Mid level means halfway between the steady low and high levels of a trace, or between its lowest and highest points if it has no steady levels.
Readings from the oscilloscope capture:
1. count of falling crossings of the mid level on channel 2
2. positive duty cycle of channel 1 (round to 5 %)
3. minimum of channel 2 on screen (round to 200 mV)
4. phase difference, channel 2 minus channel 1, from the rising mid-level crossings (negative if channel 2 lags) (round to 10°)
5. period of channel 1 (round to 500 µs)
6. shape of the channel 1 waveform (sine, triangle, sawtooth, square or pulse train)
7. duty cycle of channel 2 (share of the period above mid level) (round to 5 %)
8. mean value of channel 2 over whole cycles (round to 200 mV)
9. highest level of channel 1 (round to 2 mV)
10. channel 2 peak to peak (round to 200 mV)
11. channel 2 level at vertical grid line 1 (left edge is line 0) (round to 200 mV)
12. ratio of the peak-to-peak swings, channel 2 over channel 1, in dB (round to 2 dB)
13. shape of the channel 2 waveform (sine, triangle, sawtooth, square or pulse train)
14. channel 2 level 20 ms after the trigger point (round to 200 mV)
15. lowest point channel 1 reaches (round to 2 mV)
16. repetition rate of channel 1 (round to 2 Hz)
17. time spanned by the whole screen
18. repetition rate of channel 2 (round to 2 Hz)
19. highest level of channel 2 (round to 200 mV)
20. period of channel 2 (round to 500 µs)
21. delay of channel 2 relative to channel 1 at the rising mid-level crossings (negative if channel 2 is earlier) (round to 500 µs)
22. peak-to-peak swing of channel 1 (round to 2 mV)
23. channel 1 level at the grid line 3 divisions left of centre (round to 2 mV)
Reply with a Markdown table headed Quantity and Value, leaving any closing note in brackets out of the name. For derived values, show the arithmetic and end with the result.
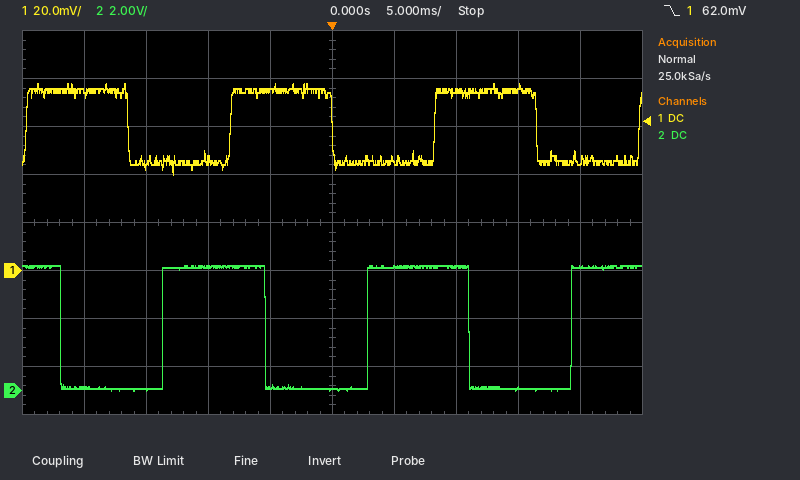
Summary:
| Quantity | Value |
|---|---|
| count of falling crossings of the mid level on channel 2 | 3 |
| positive duty cycle of channel 1 | 50 % |
| minimum of channel 2 on screen | 0.0 V |
| phase difference, channel 2 minus channel 1, from the rising mid-level crossings (negative if channel 2 lags) | −360° × (-5.5 ms) / 16.5 ms ≈ +120° |
| period of channel 1 | 16.5 ms |
| shape of the channel 1 waveform | square |
| duty cycle of channel 2 (share of the period above mid level) | 50 % |
| mean value of channel 2 over whole cycles | 0.0 V + 0.5 × (5.2 V − (0.0 V)) ≈ 2.6 V |
| highest level of channel 1 | 78 mV |
| channel 2 peak to peak | 5.2 V − (0.0 V) = 5.2 V |
| channel 2 level at vertical grid line 1 (left edge is line 0) | 200 mV |
| ratio of the peak-to-peak swings, channel 2 over channel 1, in dB | 20 log10(5.2 V / 38 mV) ≈ 42.7 dB, so 42 dB to the nearest 2 dB |
| shape of the channel 2 waveform | square |
| channel 2 level 20 ms after the trigger point | 5.2 V |
| lowest point channel 1 reaches | 40 mV |
| repetition rate of channel 1 | 1 / 16.5 ms ≈ 60.6 Hz, so 60 Hz to the nearest 2 Hz |
| time spanned by the whole screen | 50 ms |
| repetition rate of channel 2 | 1 / 16.5 ms ≈ 60.6 Hz, so 60 Hz to the nearest 2 Hz |
| highest level of channel 2 | 5.2 V |
| period of channel 2 | 16.5 ms |
| delay of channel 2 relative to channel 1 at the rising mid-level crossings (negative if channel 2 is earlier) | -5.5 ms |
| peak-to-peak swing of channel 1 | 78 mV − (40 mV) = 38 mV |
| channel 1 level at the grid line 3 divisions left of centre | 44 mV |
